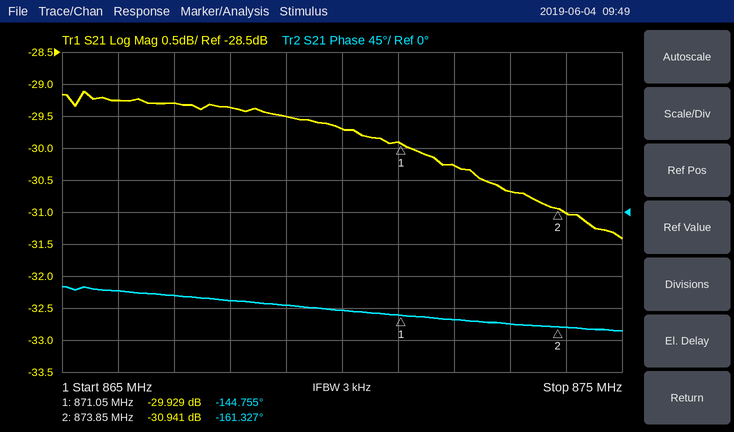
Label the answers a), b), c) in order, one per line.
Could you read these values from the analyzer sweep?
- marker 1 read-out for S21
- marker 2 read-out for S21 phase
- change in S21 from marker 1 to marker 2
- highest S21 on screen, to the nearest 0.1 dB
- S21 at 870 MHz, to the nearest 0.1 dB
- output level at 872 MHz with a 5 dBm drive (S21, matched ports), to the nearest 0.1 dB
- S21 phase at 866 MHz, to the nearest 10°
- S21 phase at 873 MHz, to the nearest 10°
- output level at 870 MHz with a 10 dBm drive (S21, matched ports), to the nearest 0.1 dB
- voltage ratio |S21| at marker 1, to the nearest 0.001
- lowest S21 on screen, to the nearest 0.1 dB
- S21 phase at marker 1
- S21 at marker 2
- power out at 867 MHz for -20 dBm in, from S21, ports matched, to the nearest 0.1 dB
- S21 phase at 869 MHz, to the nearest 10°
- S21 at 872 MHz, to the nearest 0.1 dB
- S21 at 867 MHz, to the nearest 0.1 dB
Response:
a) -29.929 dB
b) -161.327°
c) -1.012 dB
d) -29.1 dB
e) -29.7 dB
f) -25.3 dBm
g) -110°
h) -160°
i) -19.7 dBm
j) 0.032
k) -31.4 dB
l) -144.755°
m) -30.941 dB
n) -49.3 dBm
o) -130°
p) -30.3 dB
q) -29.3 dB
